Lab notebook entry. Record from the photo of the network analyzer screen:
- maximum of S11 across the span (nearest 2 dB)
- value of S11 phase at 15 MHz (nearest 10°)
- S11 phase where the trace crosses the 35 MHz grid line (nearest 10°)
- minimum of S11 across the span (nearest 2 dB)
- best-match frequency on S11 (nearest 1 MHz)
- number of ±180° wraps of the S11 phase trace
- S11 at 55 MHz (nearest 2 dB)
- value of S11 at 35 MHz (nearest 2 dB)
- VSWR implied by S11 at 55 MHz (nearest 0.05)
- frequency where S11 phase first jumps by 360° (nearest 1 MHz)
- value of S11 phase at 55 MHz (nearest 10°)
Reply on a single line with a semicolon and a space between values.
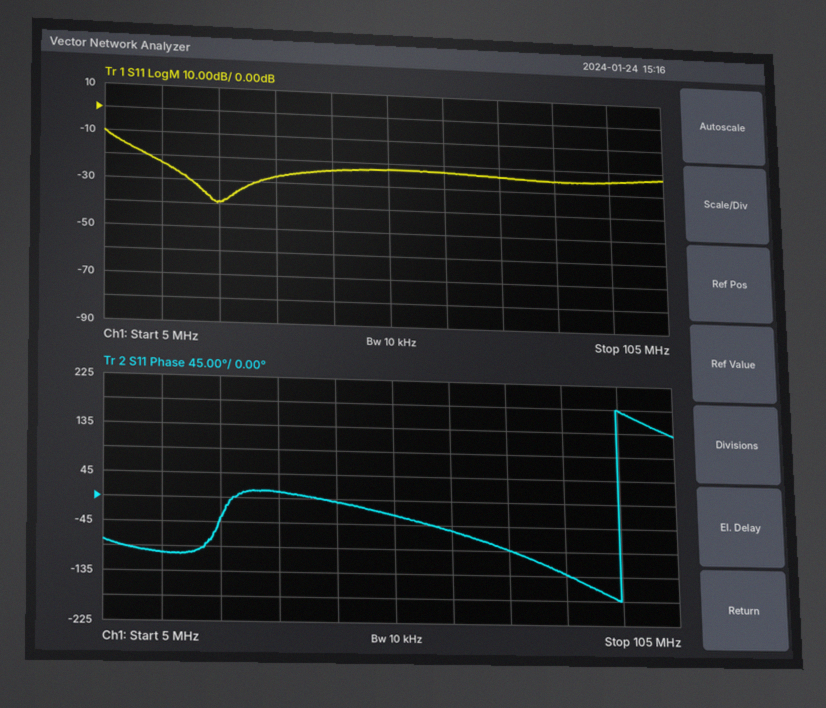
-10 dB; -100°; 10°; -40 dB; 25 MHz; 1; -22 dB; -28 dB; 1.15; 95 MHz; -30°
